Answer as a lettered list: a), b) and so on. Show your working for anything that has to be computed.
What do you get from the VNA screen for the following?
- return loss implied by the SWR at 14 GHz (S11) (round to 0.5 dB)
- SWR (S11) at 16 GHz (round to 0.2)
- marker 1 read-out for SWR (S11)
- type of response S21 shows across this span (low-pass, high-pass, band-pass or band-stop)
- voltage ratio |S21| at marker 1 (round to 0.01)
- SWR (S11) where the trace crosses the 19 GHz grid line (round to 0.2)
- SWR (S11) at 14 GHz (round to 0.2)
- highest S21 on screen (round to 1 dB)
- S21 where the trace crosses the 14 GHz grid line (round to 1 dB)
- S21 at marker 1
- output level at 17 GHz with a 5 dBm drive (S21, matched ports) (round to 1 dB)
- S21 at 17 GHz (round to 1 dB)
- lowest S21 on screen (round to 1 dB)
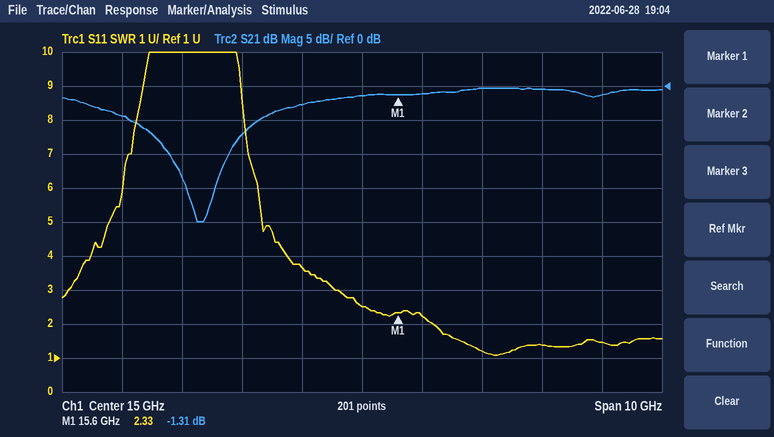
a) −20 log10((3.6 − 1)/(3.6 + 1)) ≈ 5.0 dB
b) 2.2
c) 2.33
d) band-stop
e) 10^(-1.31/20) ≈ 0.86
f) 1.4
g) 3.6
h) 0 dB
i) -3 dB
j) -1.31 dB
k) 5 dBm + (0 dB) = 5 dBm
l) 0 dB
m) -20 dB
